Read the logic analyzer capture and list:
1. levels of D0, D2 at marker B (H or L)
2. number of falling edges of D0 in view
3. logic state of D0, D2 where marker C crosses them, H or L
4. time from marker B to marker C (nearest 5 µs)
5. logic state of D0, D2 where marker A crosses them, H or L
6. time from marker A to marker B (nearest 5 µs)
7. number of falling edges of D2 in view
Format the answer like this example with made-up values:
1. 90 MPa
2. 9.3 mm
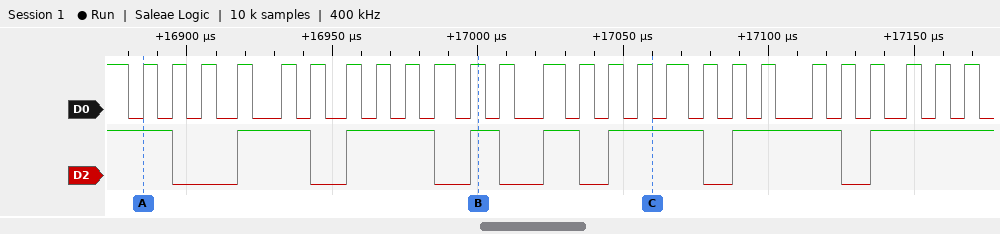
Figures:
1. D0=H, D2=H
2. 27
3. D0=L, D2=H
4. 60 µs
5. D0=H, D2=H
6. 115 µs
7. 7
